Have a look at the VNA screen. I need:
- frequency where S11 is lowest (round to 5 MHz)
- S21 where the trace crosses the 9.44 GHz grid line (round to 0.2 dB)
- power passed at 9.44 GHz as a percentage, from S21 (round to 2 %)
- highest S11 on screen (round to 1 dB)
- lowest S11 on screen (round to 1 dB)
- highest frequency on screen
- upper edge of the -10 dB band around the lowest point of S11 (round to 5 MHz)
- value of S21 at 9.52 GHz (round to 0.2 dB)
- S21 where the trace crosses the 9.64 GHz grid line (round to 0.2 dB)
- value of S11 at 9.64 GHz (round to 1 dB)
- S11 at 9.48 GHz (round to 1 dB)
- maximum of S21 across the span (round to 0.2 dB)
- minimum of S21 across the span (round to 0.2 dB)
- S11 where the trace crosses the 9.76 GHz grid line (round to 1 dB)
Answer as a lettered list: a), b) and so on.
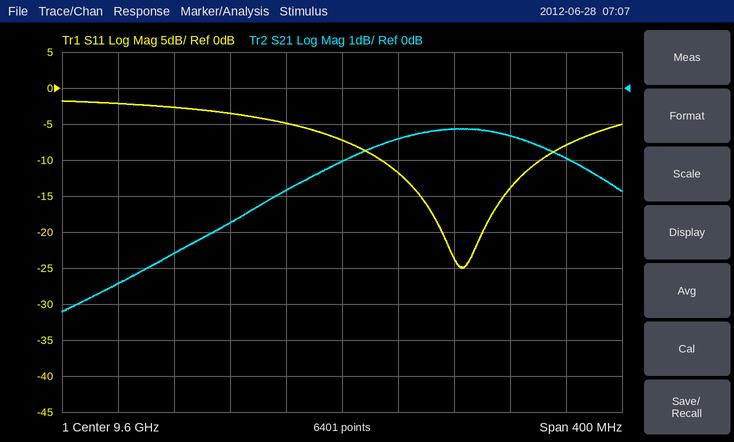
a) 9.685 GHz
b) -5.4 dB
c) 28 %
d) -2 dB
e) -25 dB
f) 9.8 GHz
g) 9.740 GHz
h) -3.8 dB
i) -1.4 dB
j) -12 dB
k) -3 dB
l) -1.2 dB
m) -6.2 dB
n) -8 dB
